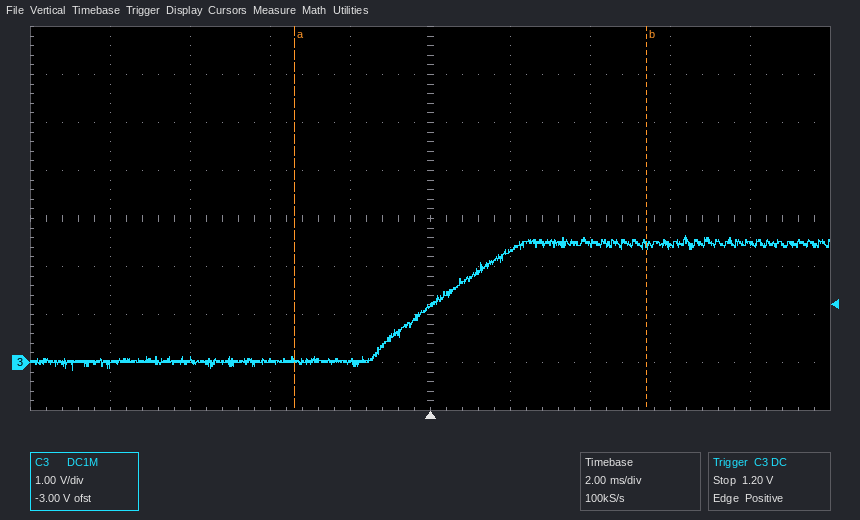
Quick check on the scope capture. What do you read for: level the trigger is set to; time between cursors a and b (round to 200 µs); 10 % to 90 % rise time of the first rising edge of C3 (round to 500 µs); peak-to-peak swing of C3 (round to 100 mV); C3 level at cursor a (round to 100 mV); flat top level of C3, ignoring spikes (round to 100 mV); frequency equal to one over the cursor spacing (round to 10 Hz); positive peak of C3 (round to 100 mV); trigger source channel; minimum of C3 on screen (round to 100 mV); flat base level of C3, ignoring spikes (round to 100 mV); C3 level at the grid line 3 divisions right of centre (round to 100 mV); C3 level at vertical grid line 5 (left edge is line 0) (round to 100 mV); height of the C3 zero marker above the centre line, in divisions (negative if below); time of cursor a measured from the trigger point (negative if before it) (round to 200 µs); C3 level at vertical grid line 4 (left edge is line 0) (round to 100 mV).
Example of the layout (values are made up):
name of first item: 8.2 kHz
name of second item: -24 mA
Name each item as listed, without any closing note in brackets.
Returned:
level the trigger is set to: 1.20 V
time between cursors a and b: 8.8 ms
10 % to 90 % rise time of the first rising edge of C3: 3.0 ms
peak-to-peak swing of C3: 2.8 V
C3 level at cursor a: 100 mV
flat top level of C3, ignoring spikes: 2.5 V
frequency equal to one over the cursor spacing: 110 Hz
positive peak of C3: 2.6 V
trigger source channel: C3
minimum of C3 on screen: -200 mV
flat base level of C3, ignoring spikes: 0.0 V
C3 level at the grid line 3 divisions right of centre: 2.4 V
C3 level at vertical grid line 5 (left edge is line 0): 1.2 V
height of the C3 zero marker above the centre line, in divisions: -3.0 div
time of cursor a measured from the trigger point (negative if before it): -3.4 ms
C3 level at vertical grid line 4 (left edge is line 0): 0.0 V
